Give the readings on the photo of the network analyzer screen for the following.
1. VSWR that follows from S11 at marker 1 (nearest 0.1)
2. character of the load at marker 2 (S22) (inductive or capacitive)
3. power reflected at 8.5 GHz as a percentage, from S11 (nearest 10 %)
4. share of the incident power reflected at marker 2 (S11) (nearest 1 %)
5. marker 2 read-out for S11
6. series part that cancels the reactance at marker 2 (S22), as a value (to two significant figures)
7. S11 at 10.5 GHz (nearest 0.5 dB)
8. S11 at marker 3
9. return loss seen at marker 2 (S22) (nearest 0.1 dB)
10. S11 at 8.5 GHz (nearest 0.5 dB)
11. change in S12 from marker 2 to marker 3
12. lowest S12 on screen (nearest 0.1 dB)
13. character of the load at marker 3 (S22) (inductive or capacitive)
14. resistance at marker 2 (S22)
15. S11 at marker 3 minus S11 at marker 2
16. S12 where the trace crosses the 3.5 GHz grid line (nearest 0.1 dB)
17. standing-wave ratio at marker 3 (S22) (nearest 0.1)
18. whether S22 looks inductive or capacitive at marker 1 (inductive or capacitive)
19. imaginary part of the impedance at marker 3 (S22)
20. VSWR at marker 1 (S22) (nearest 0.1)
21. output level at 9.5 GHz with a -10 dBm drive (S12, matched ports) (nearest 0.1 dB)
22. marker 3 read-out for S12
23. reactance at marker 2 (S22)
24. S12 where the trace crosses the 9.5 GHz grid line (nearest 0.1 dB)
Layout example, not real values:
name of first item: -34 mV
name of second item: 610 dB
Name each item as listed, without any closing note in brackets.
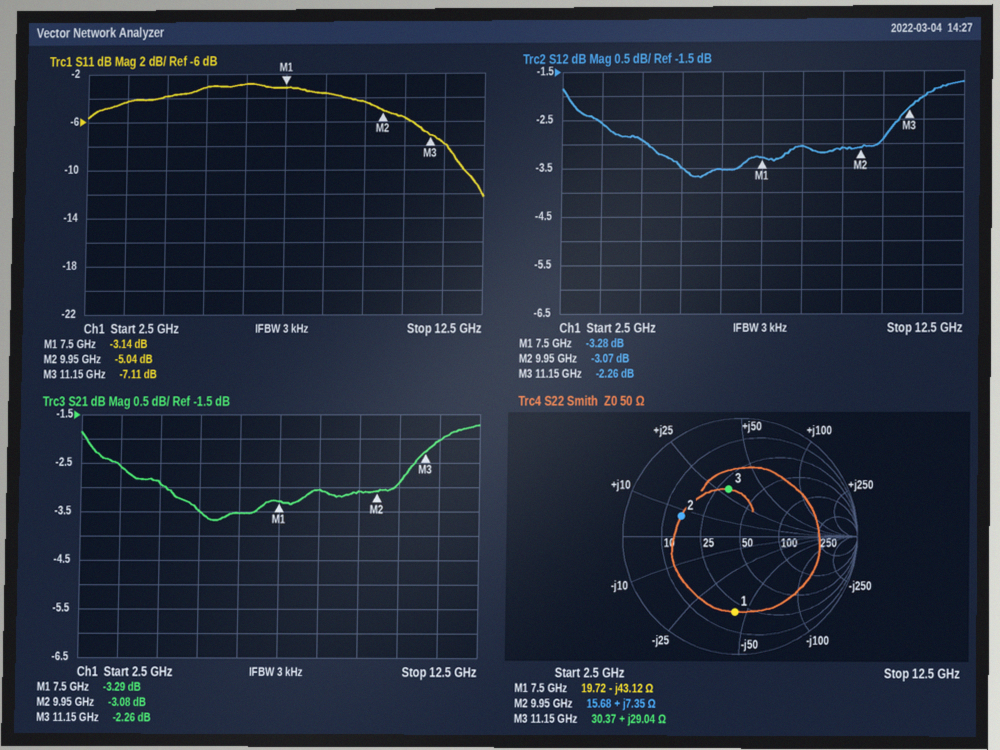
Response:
VSWR that follows from S11 at marker 1: 5.6
character of the load at marker 2 (S22): inductive
power reflected at 8.5 GHz as a percentage, from S11: 40 %
share of the incident power reflected at marker 2 (S11): 31 %
marker 2 read-out for S11: -5.04 dB
series part that cancels the reactance at marker 2 (S22), as a value: 2.2 pF
S11 at 10.5 GHz: -5.5 dB
S11 at marker 3: -7.11 dB
return loss seen at marker 2 (S22): 5.5 dB
S11 at 8.5 GHz: -3.5 dB
change in S12 from marker 2 to marker 3: 0.81 dB
lowest S12 on screen: -3.7 dB
character of the load at marker 3 (S22): inductive
resistance at marker 2: 15.68 Ω
S11 at marker 3 minus S11 at marker 2: -2.07 dB
S12 where the trace crosses the 3.5 GHz grid line: -2.6 dB
standing-wave ratio at marker 3 (S22): 2.4
whether S22 looks inductive or capacitive at marker 1: capacitive
imaginary part of the impedance at marker 3: +29.04 Ω
VSWR at marker 1 (S22): 4.6
output level at 9.5 GHz with a -10 dBm drive (S12, matched ports): -13.1 dBm
marker 3 read-out for S12: -2.26 dB
reactance at marker 2: +7.35 Ω
S12 where the trace crosses the 9.5 GHz grid line: -3.1 dB
